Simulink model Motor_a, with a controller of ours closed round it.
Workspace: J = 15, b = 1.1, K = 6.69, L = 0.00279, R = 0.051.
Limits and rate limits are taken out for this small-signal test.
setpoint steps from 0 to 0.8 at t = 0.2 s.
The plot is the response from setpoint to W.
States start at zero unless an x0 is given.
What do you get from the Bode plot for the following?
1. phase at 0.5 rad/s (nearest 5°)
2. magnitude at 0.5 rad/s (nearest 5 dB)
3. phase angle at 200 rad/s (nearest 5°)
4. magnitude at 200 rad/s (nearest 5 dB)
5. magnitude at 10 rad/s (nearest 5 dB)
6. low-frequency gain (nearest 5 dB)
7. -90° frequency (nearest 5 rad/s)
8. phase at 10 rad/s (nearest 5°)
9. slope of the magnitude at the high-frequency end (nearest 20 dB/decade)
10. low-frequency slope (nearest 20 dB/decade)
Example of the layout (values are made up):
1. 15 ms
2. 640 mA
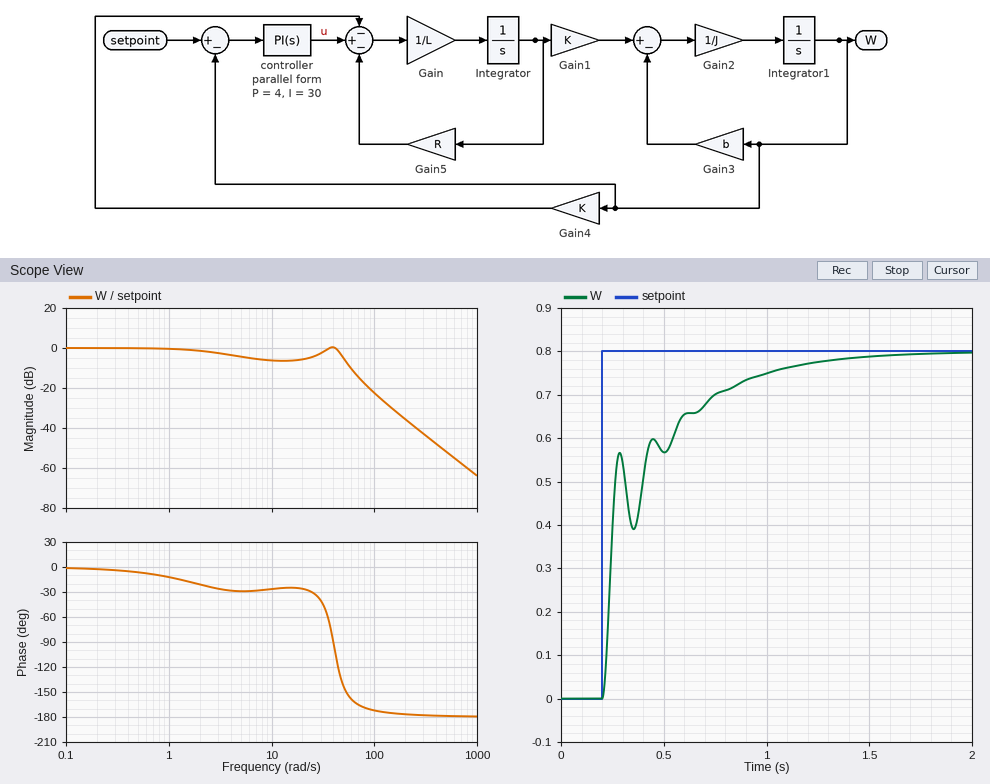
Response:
1. -5°
2. 0 dB
3. -175°
4. -35 dB
5. -5 dB
6. 0 dB
7. 40 rad/s
8. -25°
9. -40 dB/decade
10. 0 dB/decade
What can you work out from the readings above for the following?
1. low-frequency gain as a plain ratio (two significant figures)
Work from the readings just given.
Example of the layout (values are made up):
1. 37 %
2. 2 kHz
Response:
1. 1.0
